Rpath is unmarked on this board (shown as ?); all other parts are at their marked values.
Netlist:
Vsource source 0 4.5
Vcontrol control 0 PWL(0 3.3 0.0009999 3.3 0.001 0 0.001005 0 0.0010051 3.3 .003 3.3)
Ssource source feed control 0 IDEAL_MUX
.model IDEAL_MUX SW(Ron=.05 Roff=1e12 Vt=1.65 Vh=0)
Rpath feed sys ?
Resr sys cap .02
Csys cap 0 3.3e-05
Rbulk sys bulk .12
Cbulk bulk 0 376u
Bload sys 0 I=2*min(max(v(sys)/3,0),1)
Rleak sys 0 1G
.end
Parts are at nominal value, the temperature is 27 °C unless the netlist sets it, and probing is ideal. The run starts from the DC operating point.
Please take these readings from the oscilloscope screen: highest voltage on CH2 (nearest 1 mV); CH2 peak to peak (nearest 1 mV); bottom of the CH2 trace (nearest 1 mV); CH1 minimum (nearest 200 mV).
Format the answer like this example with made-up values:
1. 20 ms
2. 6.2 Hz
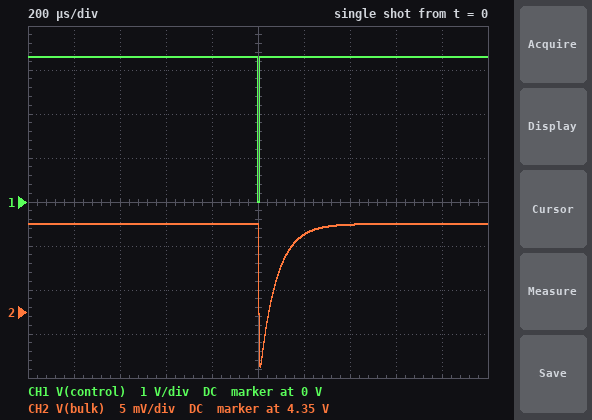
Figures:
1. 4.360 V
2. 16 mV
3. 4.344 V
4. 0 V
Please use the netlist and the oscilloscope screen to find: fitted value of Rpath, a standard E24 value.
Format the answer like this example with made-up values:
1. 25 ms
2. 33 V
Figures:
1. 0.02 Ω
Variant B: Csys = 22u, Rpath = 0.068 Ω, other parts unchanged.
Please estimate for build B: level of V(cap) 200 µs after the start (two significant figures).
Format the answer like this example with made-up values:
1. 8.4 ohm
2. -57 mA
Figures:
1. 4.3 V
